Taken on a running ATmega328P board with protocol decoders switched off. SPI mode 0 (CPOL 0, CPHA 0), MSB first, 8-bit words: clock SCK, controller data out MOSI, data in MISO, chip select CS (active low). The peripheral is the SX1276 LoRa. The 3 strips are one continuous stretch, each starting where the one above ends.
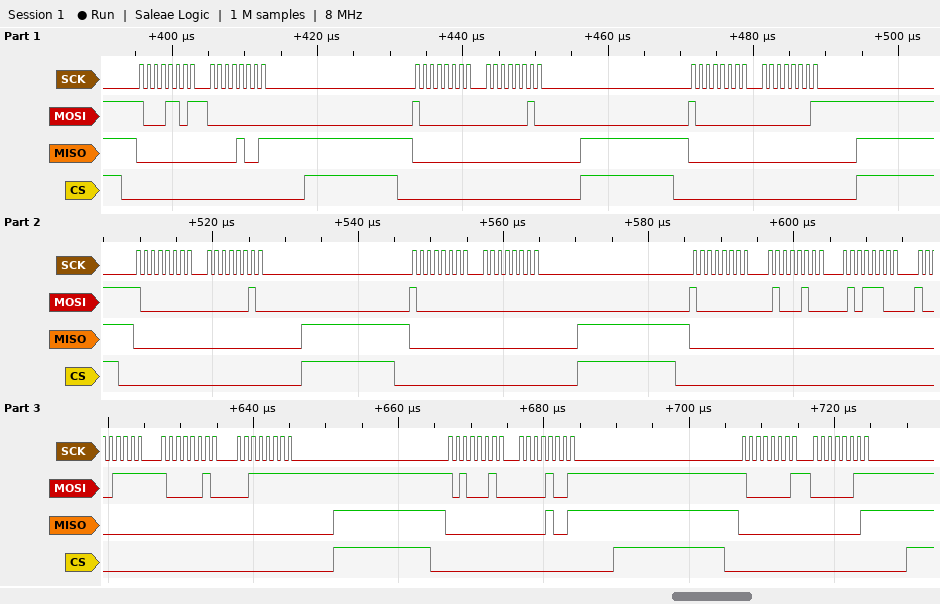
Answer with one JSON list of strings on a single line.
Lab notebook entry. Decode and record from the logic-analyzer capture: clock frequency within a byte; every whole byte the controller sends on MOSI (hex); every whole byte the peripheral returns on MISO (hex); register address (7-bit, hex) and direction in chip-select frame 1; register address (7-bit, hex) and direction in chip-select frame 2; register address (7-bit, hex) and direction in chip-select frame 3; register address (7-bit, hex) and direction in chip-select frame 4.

["1 MHz", "8D 00 80 02 80 01 80 02 80 00 80 44 5C 8F 82 3F A2 09 81 03", "00 09 00 00 00 00 00 00 00 00 00 00 00 00 00 00 00 09 00 01", "0x0D write", "0x00 write", "0x00 write", "0x00 write"]
